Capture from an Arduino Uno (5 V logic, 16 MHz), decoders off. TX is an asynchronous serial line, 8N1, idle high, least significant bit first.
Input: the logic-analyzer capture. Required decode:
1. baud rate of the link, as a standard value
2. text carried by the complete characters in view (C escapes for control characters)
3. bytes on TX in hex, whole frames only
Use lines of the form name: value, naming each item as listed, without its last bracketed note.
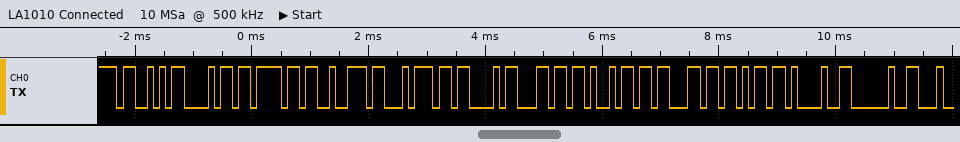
baud rate of the link, as a standard value: 9600 baud
text carried by the complete characters in view: "ShortClick! "
bytes on TX in hex, whole frames only: 53 68 6F 72 74 43 6C 69 63 6B 21 20
